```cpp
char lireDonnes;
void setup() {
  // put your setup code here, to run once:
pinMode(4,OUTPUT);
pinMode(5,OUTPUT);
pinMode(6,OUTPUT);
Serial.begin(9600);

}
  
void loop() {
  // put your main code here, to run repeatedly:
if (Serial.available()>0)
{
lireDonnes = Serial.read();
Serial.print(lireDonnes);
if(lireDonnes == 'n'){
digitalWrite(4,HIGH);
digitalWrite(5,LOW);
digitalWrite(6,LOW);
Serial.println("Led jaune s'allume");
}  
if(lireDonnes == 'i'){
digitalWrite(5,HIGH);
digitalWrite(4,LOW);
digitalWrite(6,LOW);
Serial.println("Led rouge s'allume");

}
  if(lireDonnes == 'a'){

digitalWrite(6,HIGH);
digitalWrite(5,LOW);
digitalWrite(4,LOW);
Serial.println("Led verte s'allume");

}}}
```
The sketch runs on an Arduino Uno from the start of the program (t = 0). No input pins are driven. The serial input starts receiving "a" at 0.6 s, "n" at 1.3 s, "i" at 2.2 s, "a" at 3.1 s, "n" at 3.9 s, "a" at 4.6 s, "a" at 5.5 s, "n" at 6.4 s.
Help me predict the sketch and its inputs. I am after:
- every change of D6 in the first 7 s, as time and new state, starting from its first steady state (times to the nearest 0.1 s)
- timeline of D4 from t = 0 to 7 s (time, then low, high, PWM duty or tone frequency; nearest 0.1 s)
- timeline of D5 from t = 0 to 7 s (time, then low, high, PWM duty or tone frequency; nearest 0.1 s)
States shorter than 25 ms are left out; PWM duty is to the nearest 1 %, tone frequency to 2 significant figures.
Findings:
0 s low; 0.6 s high; 1.3 s low; 3.1 s high; 3.9 s low; 4.6 s high; 6.4 s low
0 s low; 1.3 s high; 2.2 s low; 3.9 s high; 4.6 s low; 6.4 s high
0 s low; 2.2 s high; 3.1 s low
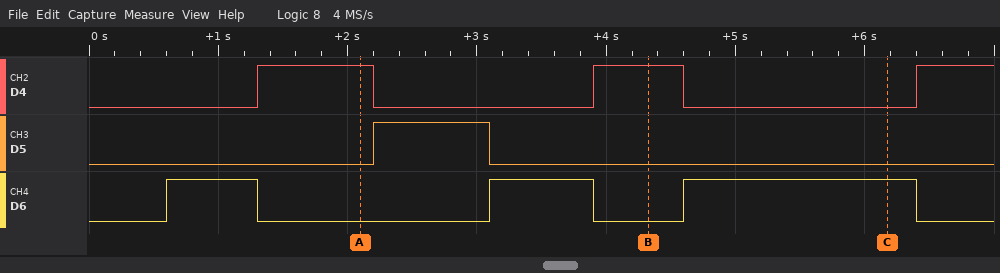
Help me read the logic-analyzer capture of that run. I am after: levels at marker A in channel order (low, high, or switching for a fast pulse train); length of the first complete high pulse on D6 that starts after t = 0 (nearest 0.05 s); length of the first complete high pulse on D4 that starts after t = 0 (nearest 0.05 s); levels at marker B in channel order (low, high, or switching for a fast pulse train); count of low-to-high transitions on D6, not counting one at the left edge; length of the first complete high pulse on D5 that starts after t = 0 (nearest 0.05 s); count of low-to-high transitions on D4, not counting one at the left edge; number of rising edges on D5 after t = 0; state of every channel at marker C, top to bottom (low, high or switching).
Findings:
D4 high, D5 low, D6 low
0.70 s
0.90 s
D4 high, D5 low, D6 low
3
0.90 s
3
1
D4 low, D5 low, D6 high
